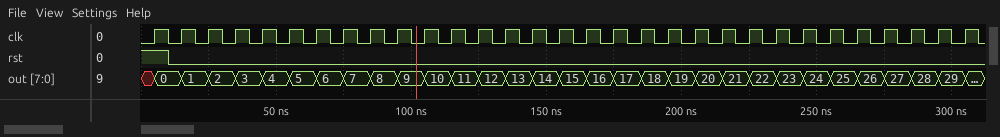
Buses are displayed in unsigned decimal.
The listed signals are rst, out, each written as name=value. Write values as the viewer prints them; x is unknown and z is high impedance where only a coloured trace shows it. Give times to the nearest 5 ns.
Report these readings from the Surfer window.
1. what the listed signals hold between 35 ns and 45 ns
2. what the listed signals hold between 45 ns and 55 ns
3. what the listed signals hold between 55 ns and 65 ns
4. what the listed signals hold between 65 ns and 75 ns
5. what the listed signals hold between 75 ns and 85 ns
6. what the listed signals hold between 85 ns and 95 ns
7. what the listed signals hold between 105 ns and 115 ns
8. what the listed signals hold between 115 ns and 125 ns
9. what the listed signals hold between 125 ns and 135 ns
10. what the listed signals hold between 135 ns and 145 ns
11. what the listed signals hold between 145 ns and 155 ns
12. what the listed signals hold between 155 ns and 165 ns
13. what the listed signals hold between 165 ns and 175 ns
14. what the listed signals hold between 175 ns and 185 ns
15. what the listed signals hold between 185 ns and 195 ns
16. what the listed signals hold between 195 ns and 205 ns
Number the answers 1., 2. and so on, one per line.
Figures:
1. rst=0, out=3
2. rst=0, out=4
3. rst=0, out=5
4. rst=0, out=6
5. rst=0, out=7
6. rst=0, out=8
7. rst=0, out=10
8. rst=0, out=11
9. rst=0, out=12
10. rst=0, out=13
11. rst=0, out=14
12. rst=0, out=15
13. rst=0, out=16
14. rst=0, out=17
15. rst=0, out=18
16. rst=0, out=19
